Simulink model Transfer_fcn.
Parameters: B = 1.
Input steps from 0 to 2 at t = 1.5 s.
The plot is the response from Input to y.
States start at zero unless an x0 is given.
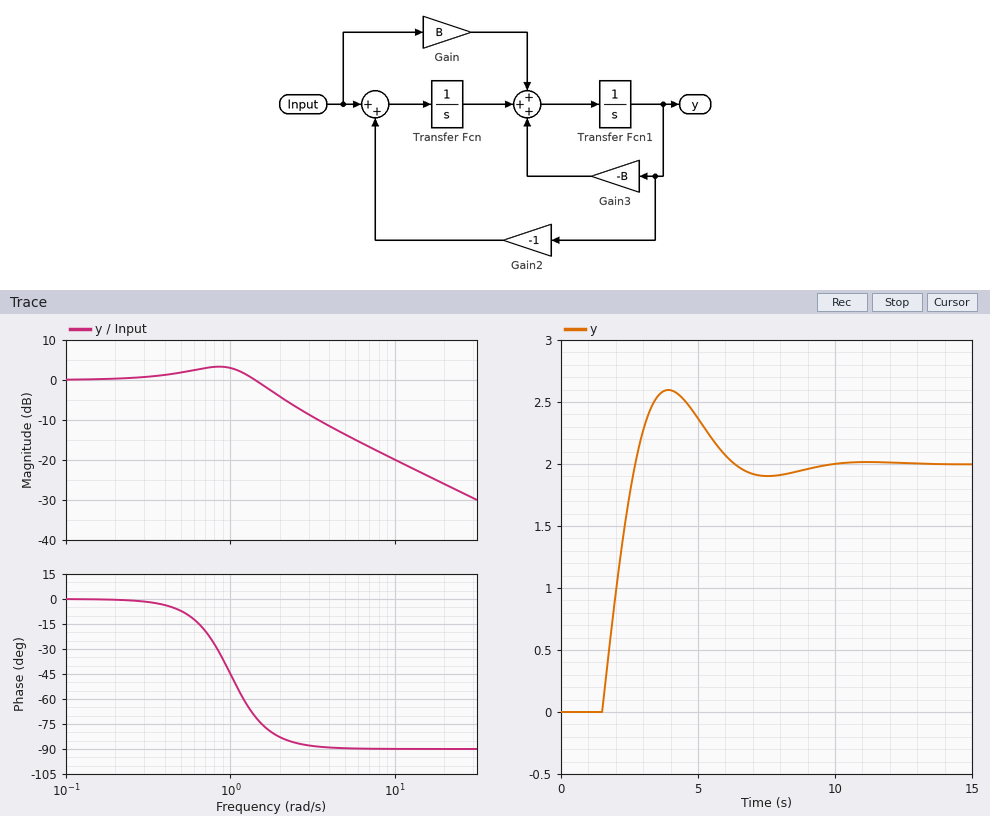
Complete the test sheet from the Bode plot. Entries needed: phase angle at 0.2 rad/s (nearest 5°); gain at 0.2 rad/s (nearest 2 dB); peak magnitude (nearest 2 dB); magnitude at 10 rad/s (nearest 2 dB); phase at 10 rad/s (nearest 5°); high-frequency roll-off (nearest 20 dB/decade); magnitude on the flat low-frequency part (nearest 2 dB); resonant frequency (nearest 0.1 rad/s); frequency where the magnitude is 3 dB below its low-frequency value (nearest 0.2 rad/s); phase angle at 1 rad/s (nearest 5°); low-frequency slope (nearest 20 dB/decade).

0°
0 dB
4 dB
-20 dB
-90°
-20 dB/decade
0 dB
0.8 rad/s
1.8 rad/s
-45°
0 dB/decade
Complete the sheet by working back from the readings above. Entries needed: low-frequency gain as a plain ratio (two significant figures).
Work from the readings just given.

1.0
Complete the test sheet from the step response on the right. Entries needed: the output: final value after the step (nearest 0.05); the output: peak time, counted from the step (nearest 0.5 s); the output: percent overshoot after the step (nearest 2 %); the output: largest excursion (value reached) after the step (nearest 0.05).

2.00
2.5 s
30 %
2.60
